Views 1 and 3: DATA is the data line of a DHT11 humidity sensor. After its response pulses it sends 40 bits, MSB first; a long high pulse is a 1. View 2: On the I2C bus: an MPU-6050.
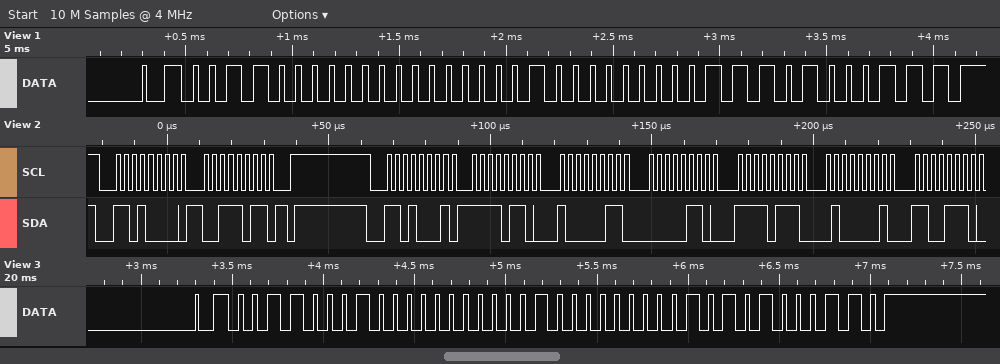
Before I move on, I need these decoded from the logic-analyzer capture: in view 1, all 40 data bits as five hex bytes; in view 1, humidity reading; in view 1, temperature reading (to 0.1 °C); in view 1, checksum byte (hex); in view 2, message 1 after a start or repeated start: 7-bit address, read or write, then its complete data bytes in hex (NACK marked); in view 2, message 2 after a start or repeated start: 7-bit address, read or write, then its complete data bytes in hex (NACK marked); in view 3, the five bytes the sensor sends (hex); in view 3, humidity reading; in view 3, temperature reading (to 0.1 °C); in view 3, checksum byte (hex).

30 00 10 07 47
48 %
16.7 °C
0x47
0x68 write: 3B
0x68 read: F6 83 06 F7 41 CE
31 00 10 05 46
49 %
16.5 °C
0x46
